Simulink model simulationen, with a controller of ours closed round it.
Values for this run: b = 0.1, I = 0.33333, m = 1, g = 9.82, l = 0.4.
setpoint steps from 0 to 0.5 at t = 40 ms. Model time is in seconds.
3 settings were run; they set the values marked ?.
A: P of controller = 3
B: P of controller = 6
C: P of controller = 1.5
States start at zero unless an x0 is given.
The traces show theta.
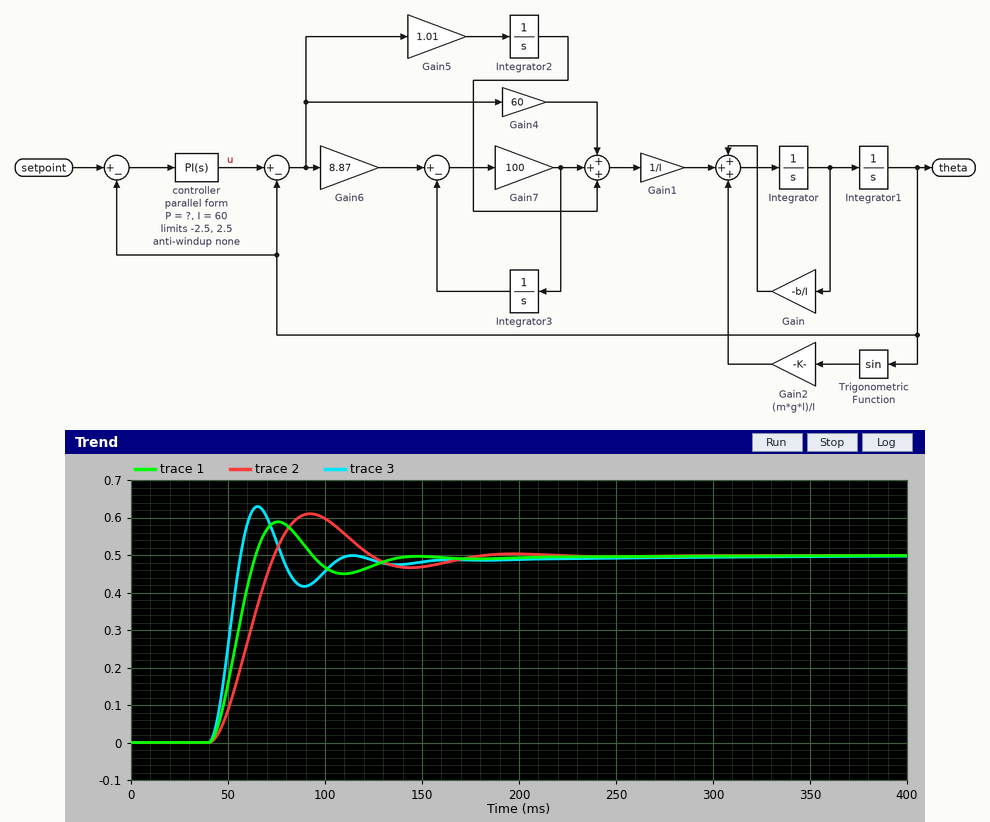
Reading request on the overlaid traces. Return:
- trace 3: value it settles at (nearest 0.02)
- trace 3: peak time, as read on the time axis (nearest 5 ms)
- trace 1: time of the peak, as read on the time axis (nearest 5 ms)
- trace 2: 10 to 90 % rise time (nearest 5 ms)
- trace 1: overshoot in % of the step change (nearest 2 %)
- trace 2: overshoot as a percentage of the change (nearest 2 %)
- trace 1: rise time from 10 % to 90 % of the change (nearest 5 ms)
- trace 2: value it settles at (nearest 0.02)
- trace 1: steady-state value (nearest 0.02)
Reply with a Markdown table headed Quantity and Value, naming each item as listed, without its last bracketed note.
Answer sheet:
| Quantity | Value |
|---|---|
| trace 3: value it settles at | 0.50 |
| trace 3: peak time, as read on the time axis | 65 ms |
| trace 1: time of the peak, as read on the time axis | 75 ms |
| trace 2: 10 to 90 % rise time | 25 ms |
| trace 1: overshoot in % of the step change | 18 % |
| trace 2: overshoot as a percentage of the change | 22 % |
| trace 1: rise time from 10 % to 90 % of the change | 15 ms |
| trace 2: value it settles at | 0.50 |
| trace 1: steady-state value | 0.50 |
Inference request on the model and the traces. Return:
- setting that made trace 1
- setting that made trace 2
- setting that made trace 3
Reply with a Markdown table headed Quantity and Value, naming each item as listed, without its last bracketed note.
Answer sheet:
| Quantity | Value |
|---|---|
| setting that made trace 1 | A |
| setting that made trace 2 | C |
| setting that made trace 3 | B |
